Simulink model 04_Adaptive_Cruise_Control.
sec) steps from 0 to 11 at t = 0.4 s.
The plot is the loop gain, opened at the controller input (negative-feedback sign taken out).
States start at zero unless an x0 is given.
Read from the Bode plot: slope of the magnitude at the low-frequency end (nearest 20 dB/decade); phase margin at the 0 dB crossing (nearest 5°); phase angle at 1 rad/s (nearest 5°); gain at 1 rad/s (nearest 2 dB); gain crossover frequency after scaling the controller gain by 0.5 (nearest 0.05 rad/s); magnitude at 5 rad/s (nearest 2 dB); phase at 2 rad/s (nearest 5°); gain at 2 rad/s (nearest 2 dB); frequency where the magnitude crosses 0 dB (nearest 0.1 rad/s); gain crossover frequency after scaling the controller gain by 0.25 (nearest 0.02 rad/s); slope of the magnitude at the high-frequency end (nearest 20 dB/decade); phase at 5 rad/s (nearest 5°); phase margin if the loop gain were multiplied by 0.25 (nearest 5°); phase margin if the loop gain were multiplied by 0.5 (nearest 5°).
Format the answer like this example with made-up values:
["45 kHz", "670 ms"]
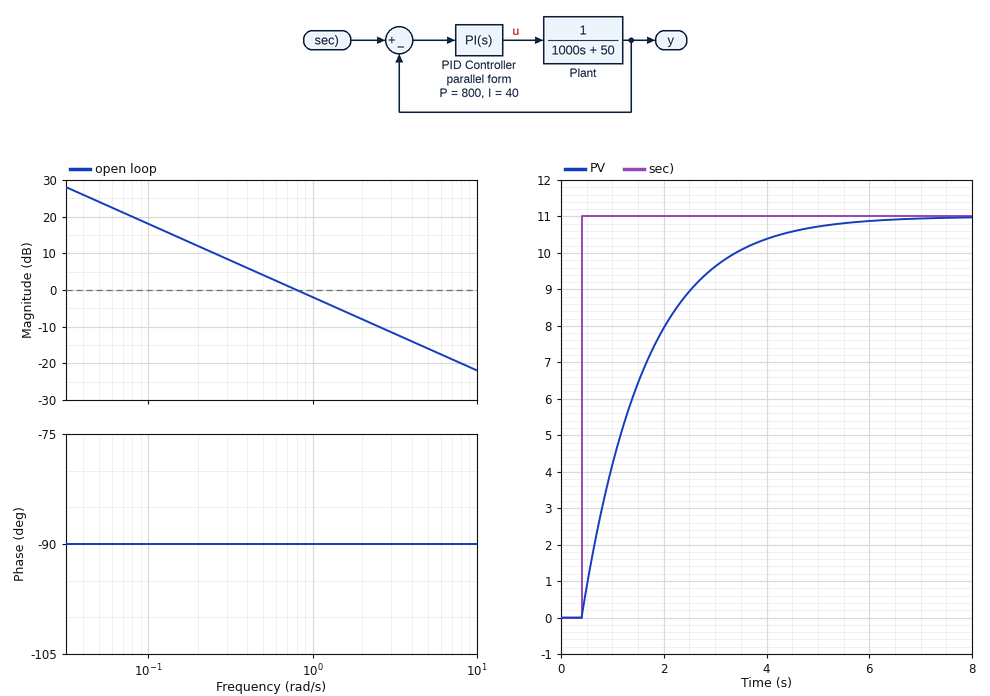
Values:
["-20 dB/decade", "90°", "-90°", "-2 dB", "0.40 rad/s", "-16 dB", "-90°", "-8 dB", "0.8 rad/s", "0.20 rad/s", "-20 dB/decade", "-90°", "90°", "90°"]
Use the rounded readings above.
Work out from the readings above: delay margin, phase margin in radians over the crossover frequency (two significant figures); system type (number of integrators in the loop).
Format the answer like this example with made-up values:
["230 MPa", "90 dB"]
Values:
["2.0 s", "1"]
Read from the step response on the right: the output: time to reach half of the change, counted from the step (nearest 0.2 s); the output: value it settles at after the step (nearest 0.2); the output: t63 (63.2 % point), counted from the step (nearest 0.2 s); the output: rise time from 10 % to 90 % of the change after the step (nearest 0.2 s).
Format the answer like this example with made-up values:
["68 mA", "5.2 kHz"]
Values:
["0.8 s", "11.0", "1.2 s", "2.8 s"]
